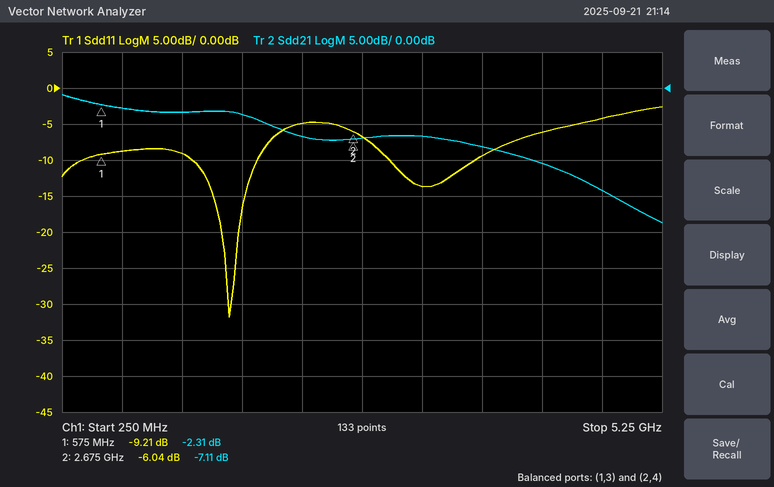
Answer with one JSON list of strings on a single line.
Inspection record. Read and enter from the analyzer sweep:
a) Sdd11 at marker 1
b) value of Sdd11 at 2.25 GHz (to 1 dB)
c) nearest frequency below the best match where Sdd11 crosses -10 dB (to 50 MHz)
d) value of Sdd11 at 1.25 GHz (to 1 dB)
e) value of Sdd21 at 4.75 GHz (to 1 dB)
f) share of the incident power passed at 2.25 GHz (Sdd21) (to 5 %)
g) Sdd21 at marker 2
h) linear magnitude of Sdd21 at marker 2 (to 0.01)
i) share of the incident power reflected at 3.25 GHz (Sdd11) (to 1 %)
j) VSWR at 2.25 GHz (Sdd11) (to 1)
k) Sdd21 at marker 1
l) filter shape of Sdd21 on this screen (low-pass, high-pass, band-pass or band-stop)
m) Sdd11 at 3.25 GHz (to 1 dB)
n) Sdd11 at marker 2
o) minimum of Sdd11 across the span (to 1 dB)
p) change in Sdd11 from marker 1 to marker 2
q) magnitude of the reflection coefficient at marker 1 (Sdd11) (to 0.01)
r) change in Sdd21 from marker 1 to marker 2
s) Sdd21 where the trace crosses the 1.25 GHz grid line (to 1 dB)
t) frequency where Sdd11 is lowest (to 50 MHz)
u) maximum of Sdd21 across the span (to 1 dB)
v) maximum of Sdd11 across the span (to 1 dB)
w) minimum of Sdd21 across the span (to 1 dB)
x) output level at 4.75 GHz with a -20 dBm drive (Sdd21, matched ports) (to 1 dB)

["-9.21 dB", "-5 dB", "1.35 GHz", "-9 dB", "-14 dB", "20 %", "-7.11 dB", "0.44", "4 %", "4", "-2.31 dB", "low-pass", "-14 dB", "-6.04 dB", "-32 dB", "3.17 dB", "0.35", "-4.80 dB", "-3 dB", "1.65 GHz", "-1 dB", "-3 dB", "-19 dB", "-34 dBm"]
